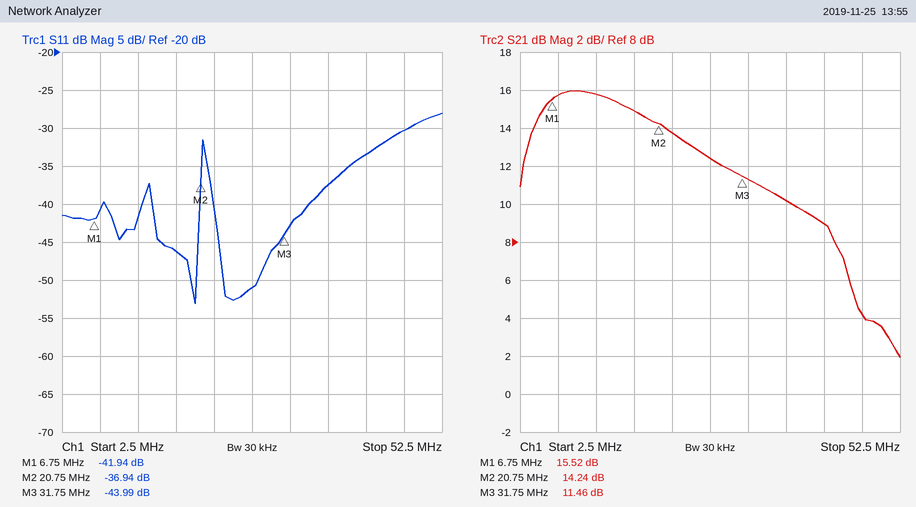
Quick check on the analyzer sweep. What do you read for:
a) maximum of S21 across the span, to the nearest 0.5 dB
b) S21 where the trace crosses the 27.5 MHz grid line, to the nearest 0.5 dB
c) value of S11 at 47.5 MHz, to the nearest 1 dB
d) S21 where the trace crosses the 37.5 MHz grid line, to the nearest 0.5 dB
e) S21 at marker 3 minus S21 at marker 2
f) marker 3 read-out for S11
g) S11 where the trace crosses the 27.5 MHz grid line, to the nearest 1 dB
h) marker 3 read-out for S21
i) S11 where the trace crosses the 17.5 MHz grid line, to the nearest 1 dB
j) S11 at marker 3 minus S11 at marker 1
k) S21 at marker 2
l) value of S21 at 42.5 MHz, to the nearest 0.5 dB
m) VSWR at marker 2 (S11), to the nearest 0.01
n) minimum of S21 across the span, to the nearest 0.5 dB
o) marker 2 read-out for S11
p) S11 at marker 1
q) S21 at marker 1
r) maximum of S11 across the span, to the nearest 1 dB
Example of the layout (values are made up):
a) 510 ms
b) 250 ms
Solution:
a) 16.0 dB
b) 12.5 dB
c) -30 dB
d) 10.0 dB
e) -2.78 dB
f) -43.99 dB
g) -51 dB
h) 11.46 dB
i) -46 dB
j) -2.05 dB
k) 14.24 dB
l) 9.0 dB
m) 1.03
n) 2.0 dB
o) -36.94 dB
p) -41.94 dB
q) 15.52 dB
r) -28 dB
